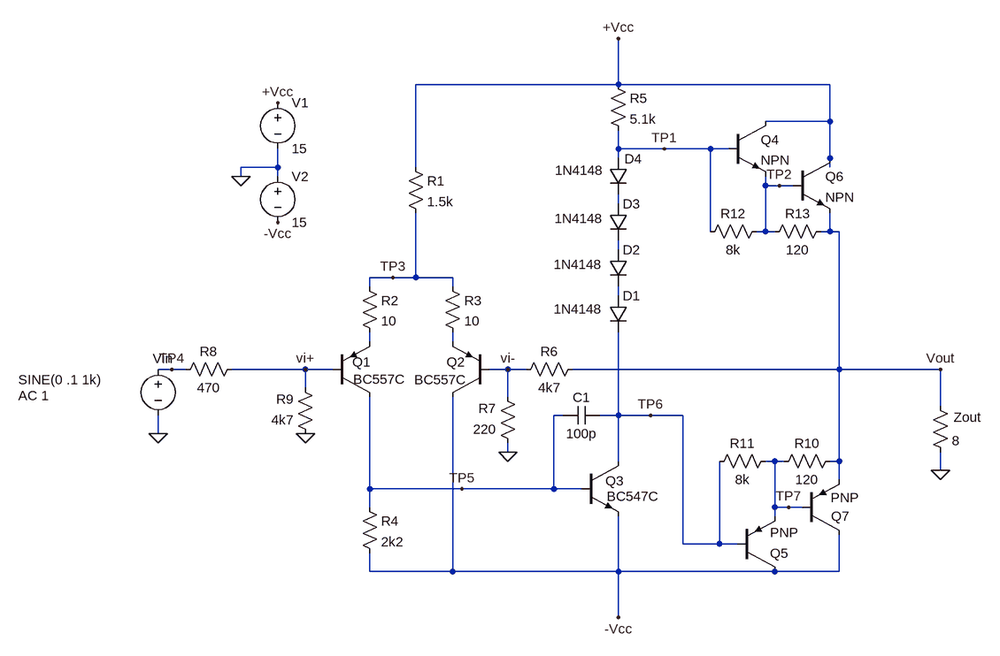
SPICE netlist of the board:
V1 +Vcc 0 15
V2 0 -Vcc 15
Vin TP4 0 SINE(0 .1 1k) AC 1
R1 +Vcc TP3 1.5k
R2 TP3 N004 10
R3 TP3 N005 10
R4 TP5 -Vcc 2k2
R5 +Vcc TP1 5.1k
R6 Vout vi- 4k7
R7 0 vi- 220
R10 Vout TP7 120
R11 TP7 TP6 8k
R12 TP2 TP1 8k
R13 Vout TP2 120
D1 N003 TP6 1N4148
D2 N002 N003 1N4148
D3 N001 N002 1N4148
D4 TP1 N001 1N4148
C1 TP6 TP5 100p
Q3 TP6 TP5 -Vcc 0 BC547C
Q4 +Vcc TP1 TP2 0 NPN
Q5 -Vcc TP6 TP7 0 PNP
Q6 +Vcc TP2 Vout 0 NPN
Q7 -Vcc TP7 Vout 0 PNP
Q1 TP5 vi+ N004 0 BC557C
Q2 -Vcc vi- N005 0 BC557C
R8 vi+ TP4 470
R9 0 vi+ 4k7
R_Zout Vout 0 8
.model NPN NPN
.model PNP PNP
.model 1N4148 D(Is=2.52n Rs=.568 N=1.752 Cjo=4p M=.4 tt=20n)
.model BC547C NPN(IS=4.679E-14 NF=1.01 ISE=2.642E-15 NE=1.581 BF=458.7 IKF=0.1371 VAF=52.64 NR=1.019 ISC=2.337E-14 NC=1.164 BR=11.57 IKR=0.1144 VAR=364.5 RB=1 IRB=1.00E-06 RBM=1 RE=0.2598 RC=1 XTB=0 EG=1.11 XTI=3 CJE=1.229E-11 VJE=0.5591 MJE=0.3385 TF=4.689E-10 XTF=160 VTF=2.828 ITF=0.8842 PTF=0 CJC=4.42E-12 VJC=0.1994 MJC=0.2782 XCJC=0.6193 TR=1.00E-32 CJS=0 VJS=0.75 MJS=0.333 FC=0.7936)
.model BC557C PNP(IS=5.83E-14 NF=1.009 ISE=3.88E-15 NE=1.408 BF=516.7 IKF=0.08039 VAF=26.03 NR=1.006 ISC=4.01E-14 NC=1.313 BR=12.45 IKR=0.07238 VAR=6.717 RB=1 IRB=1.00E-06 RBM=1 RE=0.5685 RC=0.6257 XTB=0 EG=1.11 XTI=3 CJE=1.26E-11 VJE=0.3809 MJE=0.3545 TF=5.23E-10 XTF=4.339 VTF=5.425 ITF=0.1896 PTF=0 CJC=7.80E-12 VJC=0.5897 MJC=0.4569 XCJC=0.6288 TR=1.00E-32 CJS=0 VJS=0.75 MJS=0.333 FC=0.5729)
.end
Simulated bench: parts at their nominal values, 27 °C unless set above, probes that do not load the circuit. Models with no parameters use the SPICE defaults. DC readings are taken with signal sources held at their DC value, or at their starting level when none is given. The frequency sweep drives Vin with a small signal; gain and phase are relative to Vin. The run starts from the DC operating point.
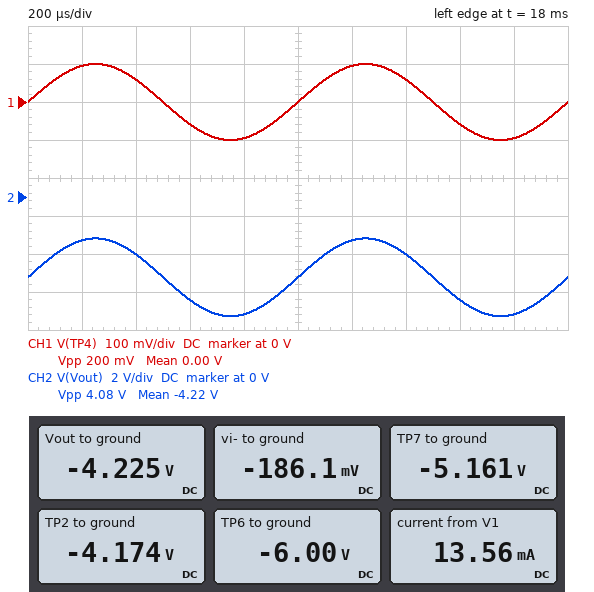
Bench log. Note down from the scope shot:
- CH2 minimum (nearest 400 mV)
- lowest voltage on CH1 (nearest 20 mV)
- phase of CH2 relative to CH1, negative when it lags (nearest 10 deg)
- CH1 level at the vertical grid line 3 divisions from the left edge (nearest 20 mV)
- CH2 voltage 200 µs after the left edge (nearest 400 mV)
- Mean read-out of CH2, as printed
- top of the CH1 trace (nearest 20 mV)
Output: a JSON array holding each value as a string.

["-6.4 V", "-100 mV", "0 deg", "-60 mV", "-2.4 V", "-4.22 V", "100 mV"]
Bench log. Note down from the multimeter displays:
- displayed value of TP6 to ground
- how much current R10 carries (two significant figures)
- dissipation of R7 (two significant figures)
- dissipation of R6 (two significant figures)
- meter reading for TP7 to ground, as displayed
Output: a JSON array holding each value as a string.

["-6.00 V", "7.8 mA", "160 µW", "3.5 mW", "-5.161 V"]
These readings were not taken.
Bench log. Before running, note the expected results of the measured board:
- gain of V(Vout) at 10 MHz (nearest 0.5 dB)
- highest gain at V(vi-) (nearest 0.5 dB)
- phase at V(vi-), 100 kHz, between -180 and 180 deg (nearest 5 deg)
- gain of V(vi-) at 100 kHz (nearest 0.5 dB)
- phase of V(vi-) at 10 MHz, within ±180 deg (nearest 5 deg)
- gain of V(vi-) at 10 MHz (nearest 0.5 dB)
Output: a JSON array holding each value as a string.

["-0.5 dB", "-1.0 dB", "-10 deg", "-1.0 dB", "95 deg", "-37.0 dB"]
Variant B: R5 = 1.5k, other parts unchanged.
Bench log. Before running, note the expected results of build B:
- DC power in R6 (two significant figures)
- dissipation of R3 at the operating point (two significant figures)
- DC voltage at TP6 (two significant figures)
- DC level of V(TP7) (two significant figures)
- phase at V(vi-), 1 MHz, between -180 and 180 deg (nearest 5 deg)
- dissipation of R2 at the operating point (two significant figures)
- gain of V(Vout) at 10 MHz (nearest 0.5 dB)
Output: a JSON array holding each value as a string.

["3.3 mW", "860 µW", "-5.9 V", "-5.1 V", "-60 deg", "1.1 µW", "0.5 dB"]
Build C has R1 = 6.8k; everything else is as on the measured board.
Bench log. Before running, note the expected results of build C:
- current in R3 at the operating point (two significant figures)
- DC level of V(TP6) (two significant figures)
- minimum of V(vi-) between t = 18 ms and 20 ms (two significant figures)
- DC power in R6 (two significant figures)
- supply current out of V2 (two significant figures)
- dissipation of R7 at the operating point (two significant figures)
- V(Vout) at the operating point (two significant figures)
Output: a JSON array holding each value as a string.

["1.8 mA", "-3.2 V", "-150 mV", "390 µW", "180 mA", "18 µW", "-1.4 V"]
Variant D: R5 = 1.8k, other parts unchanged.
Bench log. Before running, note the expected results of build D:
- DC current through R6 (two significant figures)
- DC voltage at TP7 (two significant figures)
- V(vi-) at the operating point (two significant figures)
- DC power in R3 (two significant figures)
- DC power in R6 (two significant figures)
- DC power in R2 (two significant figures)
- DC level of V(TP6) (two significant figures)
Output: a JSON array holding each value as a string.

["850 µA", "-5.1 V", "-180 mV", "860 µW", "3.4 mW", "1.1 µW", "-5.9 V"]
